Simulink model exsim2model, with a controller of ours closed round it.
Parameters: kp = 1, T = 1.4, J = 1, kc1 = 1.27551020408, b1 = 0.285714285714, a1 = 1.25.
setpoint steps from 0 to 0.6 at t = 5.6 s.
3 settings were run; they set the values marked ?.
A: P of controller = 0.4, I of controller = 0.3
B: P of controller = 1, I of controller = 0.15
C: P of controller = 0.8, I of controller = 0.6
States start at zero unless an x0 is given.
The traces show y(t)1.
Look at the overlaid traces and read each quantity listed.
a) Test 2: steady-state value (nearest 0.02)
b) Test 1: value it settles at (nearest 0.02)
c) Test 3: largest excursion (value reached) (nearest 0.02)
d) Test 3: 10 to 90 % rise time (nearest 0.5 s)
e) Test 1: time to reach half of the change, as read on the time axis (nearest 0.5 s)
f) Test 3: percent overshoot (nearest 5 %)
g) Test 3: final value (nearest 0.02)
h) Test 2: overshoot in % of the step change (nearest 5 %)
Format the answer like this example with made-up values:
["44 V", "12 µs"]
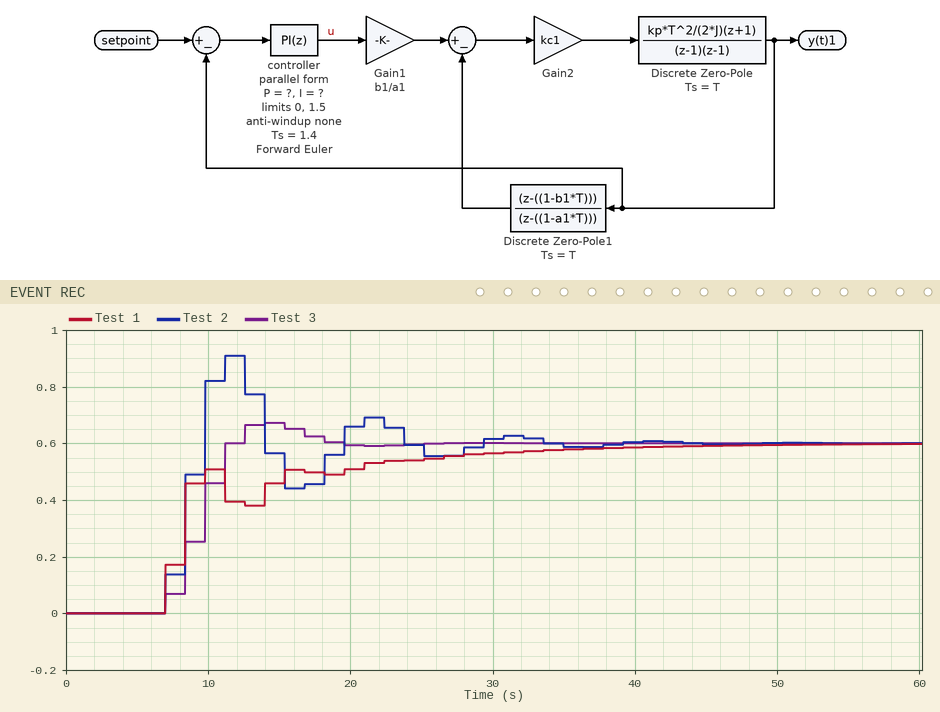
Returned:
["0.60", "0.60", "0.68", "4.0 s", "8.5 s", "10 %", "0.60", "50 %"]
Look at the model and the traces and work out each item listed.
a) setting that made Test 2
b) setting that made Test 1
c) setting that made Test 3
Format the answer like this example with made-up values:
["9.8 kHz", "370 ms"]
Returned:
["C", "B", "A"]
